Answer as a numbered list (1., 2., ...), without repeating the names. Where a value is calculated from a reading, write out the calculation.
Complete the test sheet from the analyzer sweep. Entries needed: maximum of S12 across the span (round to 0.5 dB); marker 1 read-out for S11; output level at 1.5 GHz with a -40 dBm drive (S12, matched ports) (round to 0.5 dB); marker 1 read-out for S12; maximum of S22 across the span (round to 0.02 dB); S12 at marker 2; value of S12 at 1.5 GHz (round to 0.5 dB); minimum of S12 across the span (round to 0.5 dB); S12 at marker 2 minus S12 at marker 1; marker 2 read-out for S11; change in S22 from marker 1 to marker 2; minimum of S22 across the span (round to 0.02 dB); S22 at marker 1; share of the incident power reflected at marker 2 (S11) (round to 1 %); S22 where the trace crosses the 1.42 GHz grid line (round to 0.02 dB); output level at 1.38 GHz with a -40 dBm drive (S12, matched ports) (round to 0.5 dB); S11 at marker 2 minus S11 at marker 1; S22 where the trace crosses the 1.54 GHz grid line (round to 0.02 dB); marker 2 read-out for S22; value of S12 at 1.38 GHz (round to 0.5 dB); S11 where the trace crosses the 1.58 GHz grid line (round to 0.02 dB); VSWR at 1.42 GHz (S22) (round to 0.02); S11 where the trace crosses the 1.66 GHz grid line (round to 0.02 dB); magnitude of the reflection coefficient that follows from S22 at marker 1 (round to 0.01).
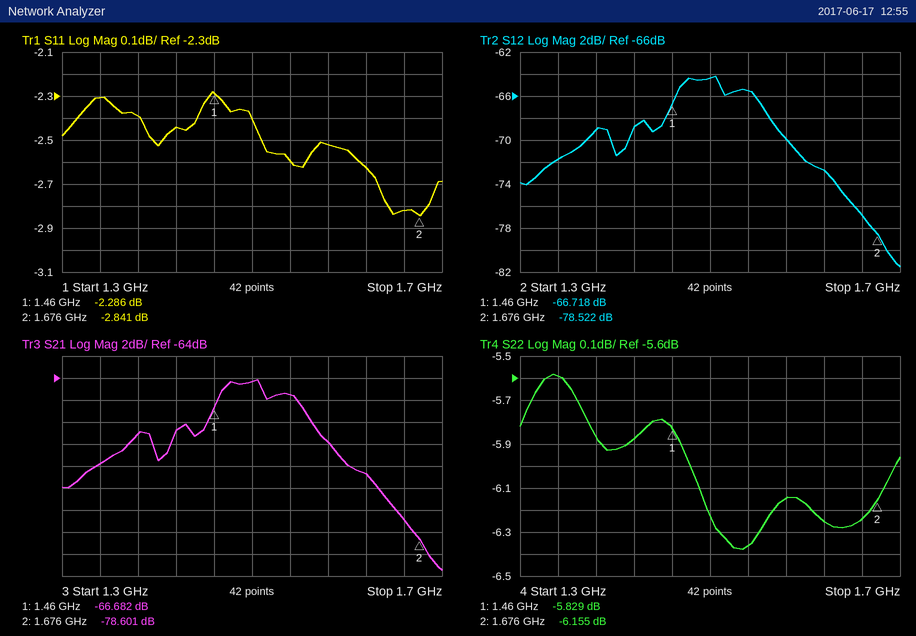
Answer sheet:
1. -64.0 dB
2. -2.286 dB
3. -40 dBm + (-64.5 dB) = -104.5 dBm
4. -66.718 dB
5. -5.58 dB
6. -78.522 dB
7. -64.5 dB
8. -81.5 dB
9. -78.522 − (-66.718) = -11.804 dB
10. -2.841 dB
11. -6.155 − (-5.829) = -0.326 dB
12. -6.38 dB
13. -5.829 dB
14. 10^(-2.841/10) ≈ 52 %
15. -5.88 dB
16. -40 dBm + (-69.0 dB) = -109.0 dBm
17. -2.841 − (-2.286) = -0.555 dB
18. -6.36 dB
19. -6.155 dB
20. -69.0 dB
21. -2.52 dB
22. |Γ| = 10^(-5.88/20) = 0.5082; VSWR = (1 + 0.5082)/(1 − 0.5082) ≈ 3.07, so 3.06 to the nearest 0.02
23. -2.82 dB
24. 10^(-5.829/20) ≈ 0.51
